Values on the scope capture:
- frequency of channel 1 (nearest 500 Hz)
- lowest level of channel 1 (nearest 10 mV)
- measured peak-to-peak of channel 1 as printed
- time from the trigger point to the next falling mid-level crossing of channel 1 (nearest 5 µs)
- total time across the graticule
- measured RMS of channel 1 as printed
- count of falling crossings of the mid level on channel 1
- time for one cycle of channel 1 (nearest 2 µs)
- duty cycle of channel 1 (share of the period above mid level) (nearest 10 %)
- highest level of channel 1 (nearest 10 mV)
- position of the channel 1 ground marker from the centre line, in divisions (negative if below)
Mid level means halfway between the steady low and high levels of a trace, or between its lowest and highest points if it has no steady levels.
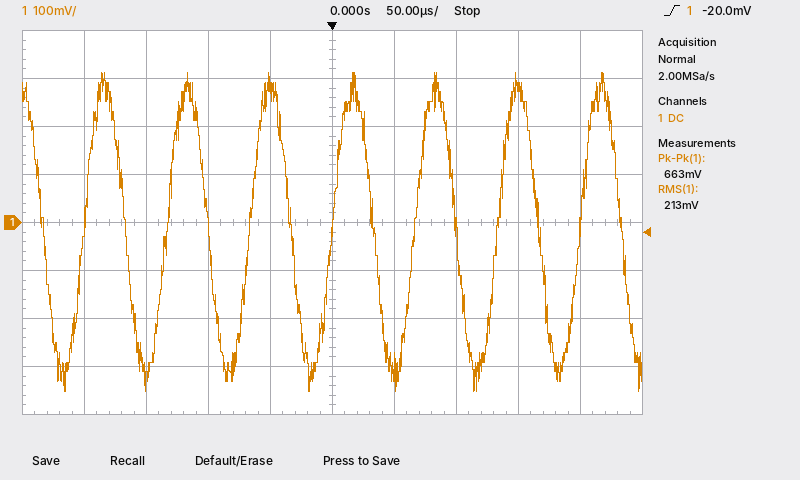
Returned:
15.0 kHz
-350 mV
663 mV
35 µs
500 µs
213 mV
8
66 µs
50 %
310 mV
0.0 div
